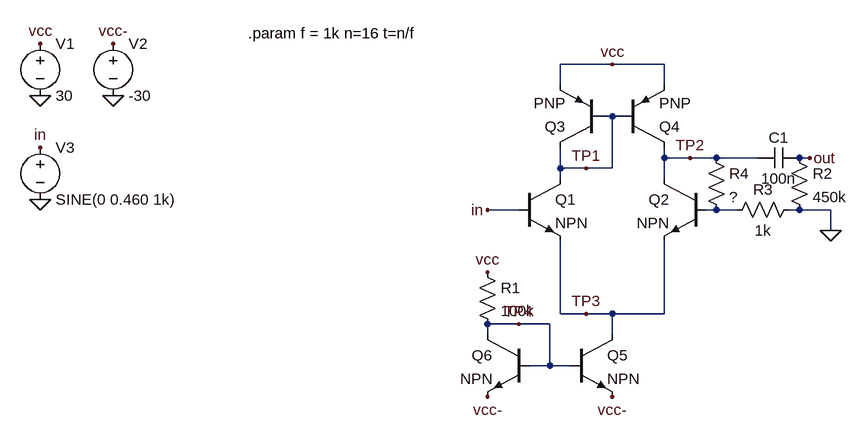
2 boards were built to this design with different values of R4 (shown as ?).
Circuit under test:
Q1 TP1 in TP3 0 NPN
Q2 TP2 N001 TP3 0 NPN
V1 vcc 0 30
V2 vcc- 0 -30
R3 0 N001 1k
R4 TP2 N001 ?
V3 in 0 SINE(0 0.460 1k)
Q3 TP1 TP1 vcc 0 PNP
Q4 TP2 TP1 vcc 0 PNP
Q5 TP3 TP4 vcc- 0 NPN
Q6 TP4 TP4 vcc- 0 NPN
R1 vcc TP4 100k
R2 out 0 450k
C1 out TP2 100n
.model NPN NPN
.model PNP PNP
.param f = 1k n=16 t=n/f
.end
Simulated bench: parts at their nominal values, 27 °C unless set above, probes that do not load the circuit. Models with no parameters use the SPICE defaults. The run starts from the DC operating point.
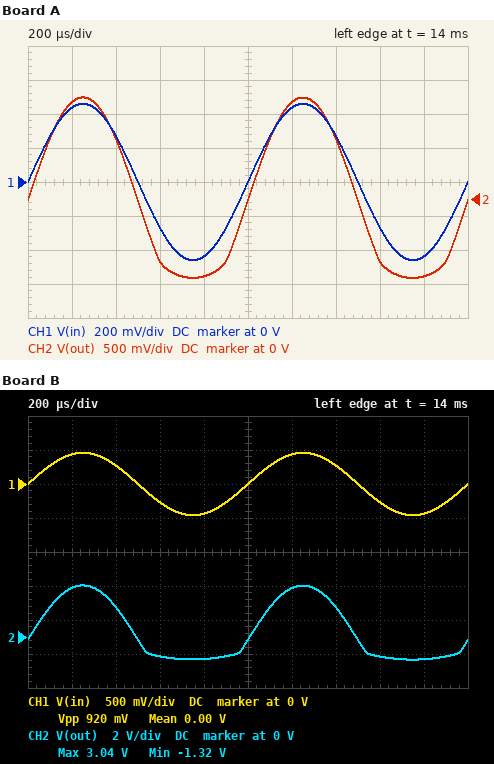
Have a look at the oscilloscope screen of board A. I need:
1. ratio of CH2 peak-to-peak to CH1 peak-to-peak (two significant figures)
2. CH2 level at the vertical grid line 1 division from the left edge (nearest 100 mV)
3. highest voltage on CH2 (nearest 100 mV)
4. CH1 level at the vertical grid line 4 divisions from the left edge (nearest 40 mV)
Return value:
2.9
1.4 V
1.5 V
-440 mV
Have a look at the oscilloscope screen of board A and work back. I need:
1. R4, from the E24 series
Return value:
2.7 kΩ
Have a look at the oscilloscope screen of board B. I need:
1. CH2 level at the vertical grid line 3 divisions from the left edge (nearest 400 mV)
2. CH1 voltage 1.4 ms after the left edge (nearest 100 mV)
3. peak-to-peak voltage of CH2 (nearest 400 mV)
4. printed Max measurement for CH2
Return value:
-1.2 V
300 mV
4.4 V
3.04 V
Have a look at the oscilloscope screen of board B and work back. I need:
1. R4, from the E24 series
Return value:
6.8 kΩ
